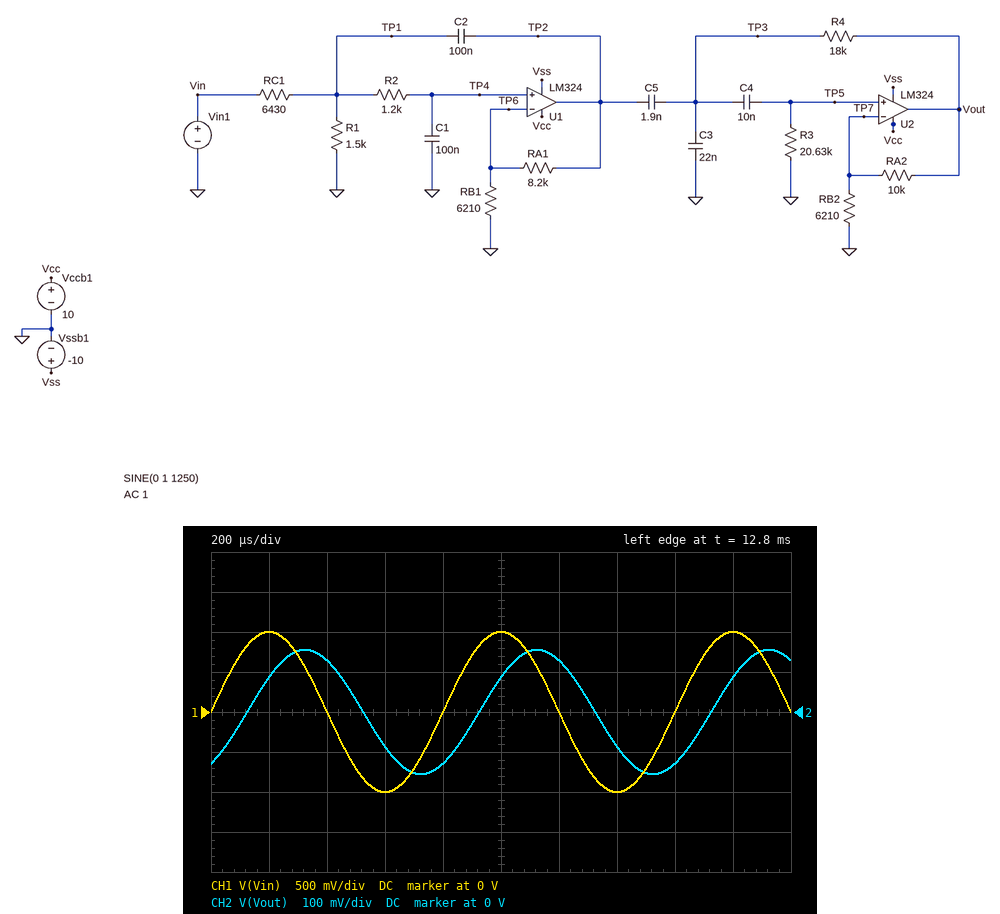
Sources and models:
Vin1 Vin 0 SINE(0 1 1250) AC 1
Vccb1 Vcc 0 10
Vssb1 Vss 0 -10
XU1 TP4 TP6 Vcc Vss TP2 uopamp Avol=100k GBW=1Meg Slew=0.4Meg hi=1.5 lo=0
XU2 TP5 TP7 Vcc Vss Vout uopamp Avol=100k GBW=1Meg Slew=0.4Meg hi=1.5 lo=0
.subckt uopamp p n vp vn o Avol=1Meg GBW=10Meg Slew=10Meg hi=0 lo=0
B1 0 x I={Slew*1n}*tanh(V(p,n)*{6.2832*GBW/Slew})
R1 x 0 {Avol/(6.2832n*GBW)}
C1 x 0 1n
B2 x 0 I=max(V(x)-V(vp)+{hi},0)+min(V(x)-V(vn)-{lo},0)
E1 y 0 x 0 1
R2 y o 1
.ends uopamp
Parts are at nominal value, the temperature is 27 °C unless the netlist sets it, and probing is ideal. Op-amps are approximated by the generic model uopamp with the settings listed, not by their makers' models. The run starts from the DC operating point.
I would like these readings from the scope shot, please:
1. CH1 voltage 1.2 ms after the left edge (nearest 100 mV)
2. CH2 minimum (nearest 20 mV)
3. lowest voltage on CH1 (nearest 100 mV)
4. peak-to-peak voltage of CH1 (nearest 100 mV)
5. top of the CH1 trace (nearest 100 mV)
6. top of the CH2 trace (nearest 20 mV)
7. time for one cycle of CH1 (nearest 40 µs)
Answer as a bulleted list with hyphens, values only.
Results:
- 0 V
- -160 mV
- -1.0 V
- 2.0 V
- 1.0 V
- 160 mV
- 800 µs
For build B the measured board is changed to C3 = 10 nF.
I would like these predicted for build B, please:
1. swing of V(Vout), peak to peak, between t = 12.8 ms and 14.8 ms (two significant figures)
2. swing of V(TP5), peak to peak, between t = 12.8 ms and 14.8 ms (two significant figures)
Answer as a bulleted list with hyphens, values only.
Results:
- 860 mV
- 330 mV
